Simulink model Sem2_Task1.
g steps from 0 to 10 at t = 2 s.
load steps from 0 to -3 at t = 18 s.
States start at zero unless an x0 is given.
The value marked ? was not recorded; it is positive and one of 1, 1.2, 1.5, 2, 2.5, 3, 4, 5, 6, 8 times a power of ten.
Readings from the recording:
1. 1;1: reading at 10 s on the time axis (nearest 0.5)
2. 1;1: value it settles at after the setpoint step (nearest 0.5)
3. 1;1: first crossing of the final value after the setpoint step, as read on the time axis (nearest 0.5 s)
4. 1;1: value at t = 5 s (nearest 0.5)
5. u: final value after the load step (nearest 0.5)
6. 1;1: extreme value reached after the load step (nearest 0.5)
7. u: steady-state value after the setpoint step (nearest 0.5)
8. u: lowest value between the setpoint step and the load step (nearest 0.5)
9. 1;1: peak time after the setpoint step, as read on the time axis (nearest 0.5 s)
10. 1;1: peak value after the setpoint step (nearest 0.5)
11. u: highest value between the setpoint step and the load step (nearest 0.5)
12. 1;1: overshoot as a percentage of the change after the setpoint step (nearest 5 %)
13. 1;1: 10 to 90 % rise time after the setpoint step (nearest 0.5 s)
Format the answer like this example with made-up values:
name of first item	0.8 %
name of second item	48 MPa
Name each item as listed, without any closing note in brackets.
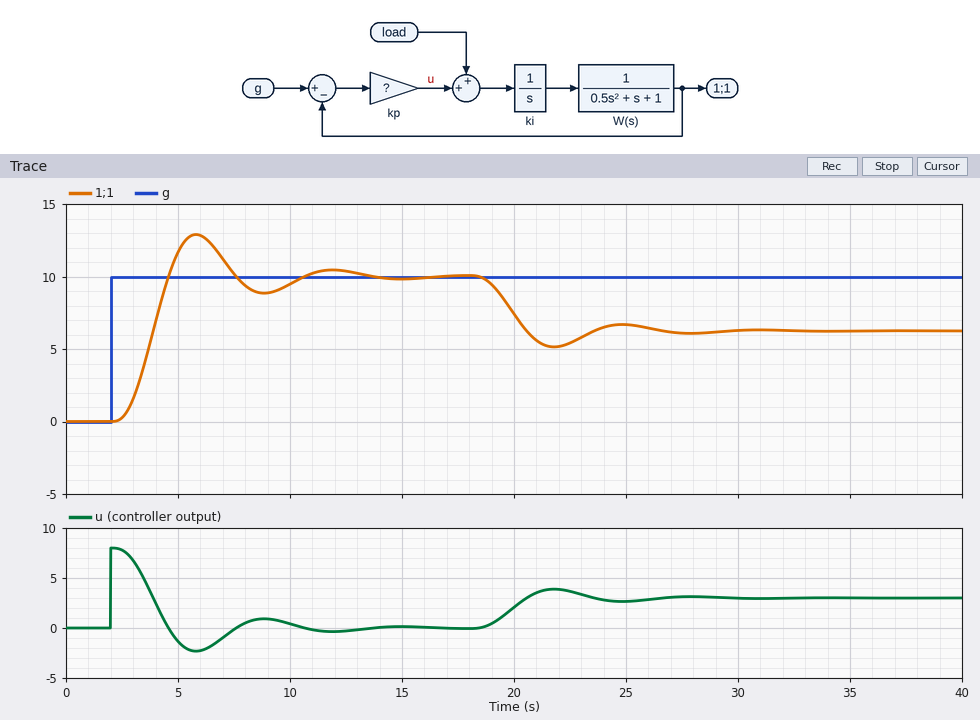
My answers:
1;1: reading at 10 s on the time axis	9.5
1;1: value it settles at after the setpoint step	10.0
1;1: first crossing of the final value after the setpoint step, as read on the time axis	4.5 s
1;1: value at t = 5 s	11.5
u: final value after the load step	3.0
1;1: extreme value reached after the load step	5.0
u: steady-state value after the setpoint step	0.0
u: lowest value between the setpoint step and the load step	-2.5
1;1: peak time after the setpoint step, as read on the time axis	6.0 s
1;1: peak value after the setpoint step	13.0
u: highest value between the setpoint step and the load step	8.0
1;1: overshoot as a percentage of the change after the setpoint step	30 %
1;1: 10 to 90 % rise time after the setpoint step	1.5 s
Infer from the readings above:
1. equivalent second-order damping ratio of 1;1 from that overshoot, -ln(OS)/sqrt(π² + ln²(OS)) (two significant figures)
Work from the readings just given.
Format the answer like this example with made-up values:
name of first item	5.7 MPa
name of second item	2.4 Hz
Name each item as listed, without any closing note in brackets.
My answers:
equivalent second-order damping ratio of 1;1 from that overshoot, -ln(OS)/sqrt(π² + ln²(OS))	0.36
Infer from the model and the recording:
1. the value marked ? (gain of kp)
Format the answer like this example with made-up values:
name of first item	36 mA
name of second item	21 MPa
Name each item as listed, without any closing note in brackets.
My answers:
the value marked ?	0.8
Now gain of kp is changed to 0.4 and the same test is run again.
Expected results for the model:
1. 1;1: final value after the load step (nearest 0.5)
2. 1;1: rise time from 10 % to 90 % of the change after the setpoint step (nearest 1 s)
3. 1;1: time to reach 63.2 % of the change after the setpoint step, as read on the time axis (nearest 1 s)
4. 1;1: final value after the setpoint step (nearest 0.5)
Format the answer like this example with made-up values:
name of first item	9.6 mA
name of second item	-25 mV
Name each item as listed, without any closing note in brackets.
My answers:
1;1: final value after the load step	2.5
1;1: rise time from 10 % to 90 % of the change after the setpoint step	3 s
1;1: time to reach 63.2 % of the change after the setpoint step, as read on the time axis	5 s
1;1: final value after the setpoint step	10.0
